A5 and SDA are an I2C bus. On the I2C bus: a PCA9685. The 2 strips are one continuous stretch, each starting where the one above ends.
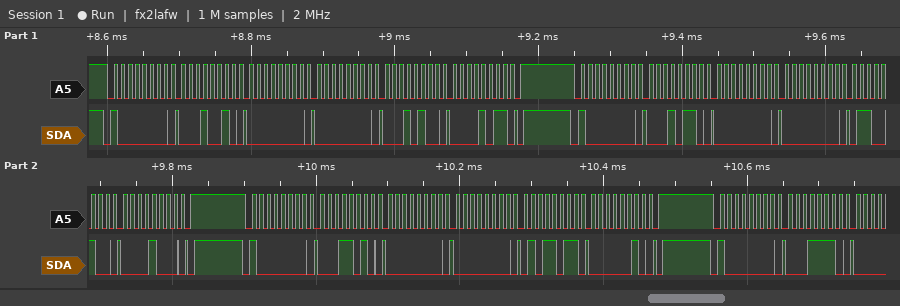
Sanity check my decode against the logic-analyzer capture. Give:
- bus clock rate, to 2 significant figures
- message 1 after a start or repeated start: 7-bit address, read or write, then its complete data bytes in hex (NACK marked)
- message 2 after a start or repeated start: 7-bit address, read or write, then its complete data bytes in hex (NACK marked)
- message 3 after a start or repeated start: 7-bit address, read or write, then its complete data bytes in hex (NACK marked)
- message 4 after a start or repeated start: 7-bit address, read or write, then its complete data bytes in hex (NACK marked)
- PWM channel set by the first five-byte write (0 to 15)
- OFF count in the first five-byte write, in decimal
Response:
100 kHz
0x40 write: 12 00 00 14 0B
0x40 write: 16 00 00 64 08
0x40 write: 1A 00 00 5B 02
0x40 write: 1E
3
2836
